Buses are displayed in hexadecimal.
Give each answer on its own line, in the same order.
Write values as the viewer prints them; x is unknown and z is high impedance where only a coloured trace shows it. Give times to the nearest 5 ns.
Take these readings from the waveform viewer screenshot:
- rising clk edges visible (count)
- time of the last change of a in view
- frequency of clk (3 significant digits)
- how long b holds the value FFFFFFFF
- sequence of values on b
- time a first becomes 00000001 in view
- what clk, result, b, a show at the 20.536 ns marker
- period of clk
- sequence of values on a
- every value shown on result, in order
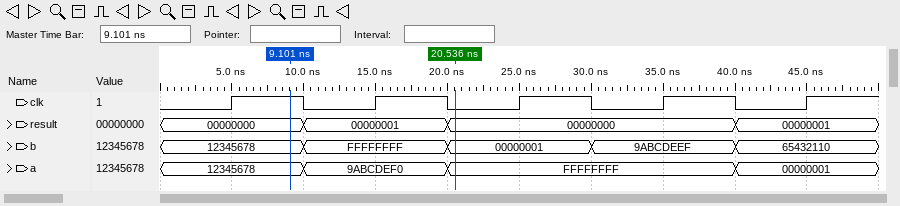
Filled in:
5
40 ns
100 MHz
10 ns
12345678, FFFFFFFF, 00000001, 9ABCDEEF, 65432110
40 ns
clk=0, result=00000000, b=00000001, a=FFFFFFFF
10 ns
12345678, 9ABCDEF0, FFFFFFFF, 00000001
00000000, 00000001, 00000000, 00000001
